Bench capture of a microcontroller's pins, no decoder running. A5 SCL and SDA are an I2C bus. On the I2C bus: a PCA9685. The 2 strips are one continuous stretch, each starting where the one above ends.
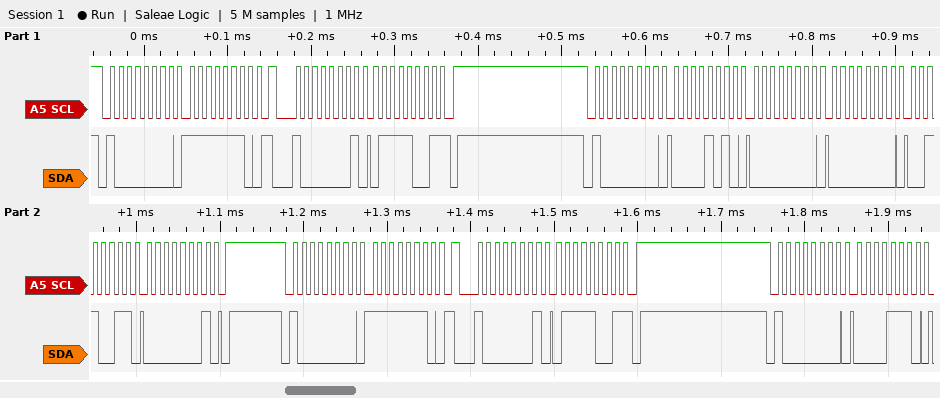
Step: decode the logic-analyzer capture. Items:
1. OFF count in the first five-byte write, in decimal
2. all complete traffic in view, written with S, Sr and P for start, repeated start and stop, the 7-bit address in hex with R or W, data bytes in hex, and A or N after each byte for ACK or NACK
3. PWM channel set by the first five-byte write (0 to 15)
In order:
307
S 40W A FE A Sr 40R A 79 N P S 40W A 0A A 00 A 00 A 33 A 01 A P S 40W A FE A Sr 40R A 79 N P S 40W A 0E A
1
